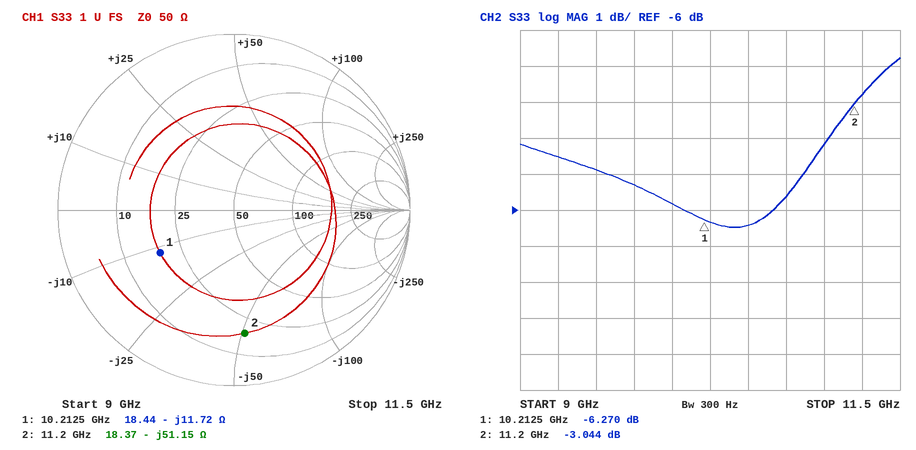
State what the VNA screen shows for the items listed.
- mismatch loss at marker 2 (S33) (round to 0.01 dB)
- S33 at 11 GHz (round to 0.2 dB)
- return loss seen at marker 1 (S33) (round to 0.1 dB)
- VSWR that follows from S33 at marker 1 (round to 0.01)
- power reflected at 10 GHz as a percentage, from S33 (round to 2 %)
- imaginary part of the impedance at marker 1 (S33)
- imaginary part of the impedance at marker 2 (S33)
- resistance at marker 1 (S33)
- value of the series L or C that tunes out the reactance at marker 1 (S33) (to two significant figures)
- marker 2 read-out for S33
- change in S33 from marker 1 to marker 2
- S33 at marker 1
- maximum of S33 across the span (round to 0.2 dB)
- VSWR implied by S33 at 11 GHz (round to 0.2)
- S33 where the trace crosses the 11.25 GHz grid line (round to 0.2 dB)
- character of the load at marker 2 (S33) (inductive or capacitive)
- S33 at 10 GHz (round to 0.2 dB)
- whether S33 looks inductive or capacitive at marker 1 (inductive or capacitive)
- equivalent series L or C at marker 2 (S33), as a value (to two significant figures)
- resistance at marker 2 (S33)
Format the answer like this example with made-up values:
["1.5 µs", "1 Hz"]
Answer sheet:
["2.98 dB", "-4.2 dB", "6.3 dB", "2.89", "26 %", "-11.72 Ω", "-51.15 Ω", "18.44 Ω", "180 pH", "-3.044 dB", "3.226 dB", "-6.270 dB", "-1.8 dB", "4.2", "-2.8 dB", "capacitive", "-5.8 dB", "capacitive", "280 fF", "18.37 Ω"]
